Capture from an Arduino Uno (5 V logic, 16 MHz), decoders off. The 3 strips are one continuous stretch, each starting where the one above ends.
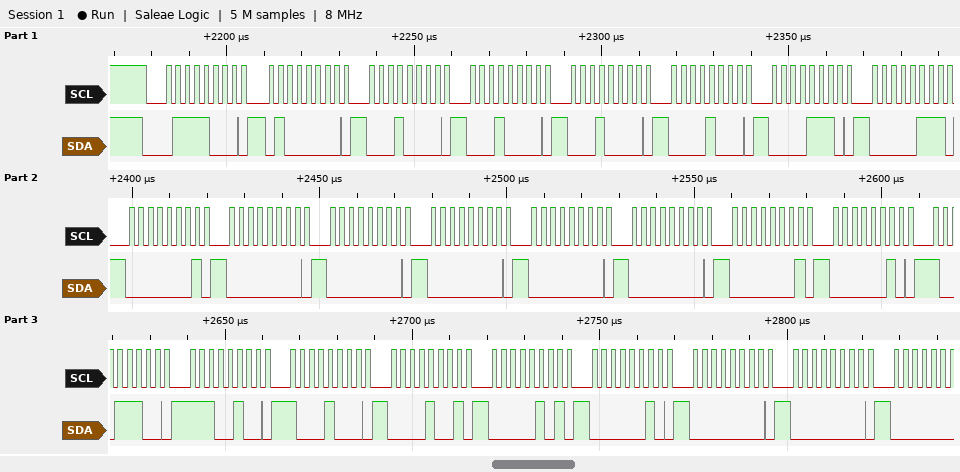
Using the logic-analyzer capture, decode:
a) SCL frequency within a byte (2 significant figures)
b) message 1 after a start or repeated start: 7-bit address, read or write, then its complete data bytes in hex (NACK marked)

400 kHz
0x3C write: 40 10 10 10 08 0E 07 01 00 00 00 00 00 01 02 9C E4 88 09 05 02 00 00
